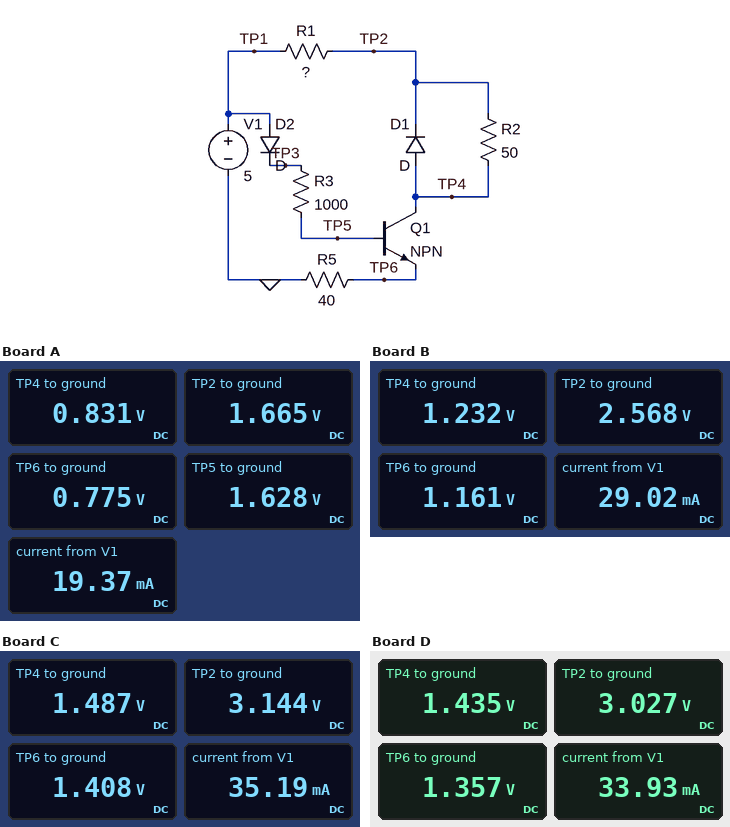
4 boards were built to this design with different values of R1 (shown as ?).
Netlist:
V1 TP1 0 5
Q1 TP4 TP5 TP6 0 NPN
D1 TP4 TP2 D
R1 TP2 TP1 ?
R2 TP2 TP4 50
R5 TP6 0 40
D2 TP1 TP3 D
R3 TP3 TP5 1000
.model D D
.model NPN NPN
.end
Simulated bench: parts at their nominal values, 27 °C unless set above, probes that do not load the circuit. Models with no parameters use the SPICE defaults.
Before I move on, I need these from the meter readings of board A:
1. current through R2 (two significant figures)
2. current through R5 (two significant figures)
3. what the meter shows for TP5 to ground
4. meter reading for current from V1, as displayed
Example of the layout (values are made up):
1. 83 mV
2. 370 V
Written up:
1. 17 mA
2. 19 mA
3. 1.628 V
4. 19.37 mA
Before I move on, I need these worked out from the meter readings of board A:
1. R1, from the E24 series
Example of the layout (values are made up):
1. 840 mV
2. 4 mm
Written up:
1. 200 Ω
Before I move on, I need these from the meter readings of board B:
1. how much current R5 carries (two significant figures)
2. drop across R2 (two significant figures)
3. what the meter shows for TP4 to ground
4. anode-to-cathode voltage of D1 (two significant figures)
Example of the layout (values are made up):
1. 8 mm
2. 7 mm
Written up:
1. 29 mA
2. 1.3 V
3. 1.232 V
4. -1.3 V
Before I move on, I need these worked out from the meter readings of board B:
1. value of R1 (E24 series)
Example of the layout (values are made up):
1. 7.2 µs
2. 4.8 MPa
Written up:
1. 91 Ω
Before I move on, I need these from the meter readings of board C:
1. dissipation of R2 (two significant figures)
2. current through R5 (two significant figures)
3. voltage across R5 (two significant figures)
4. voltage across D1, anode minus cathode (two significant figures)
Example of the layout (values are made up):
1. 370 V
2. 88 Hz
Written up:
1. 55 mW
2. 35 mA
3. 1.4 V
4. -1.7 V
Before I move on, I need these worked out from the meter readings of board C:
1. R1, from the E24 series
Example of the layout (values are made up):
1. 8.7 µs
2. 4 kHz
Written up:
1. 56 Ω
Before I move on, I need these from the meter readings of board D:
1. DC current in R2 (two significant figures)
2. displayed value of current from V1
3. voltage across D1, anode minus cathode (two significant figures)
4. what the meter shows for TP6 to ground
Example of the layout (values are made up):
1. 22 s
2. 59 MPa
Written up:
1. 32 mA
2. 33.93 mA
3. -1.6 V
4. 1.357 V
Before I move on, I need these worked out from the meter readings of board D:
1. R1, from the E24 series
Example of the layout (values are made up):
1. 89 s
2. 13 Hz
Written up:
1. 62 Ω
